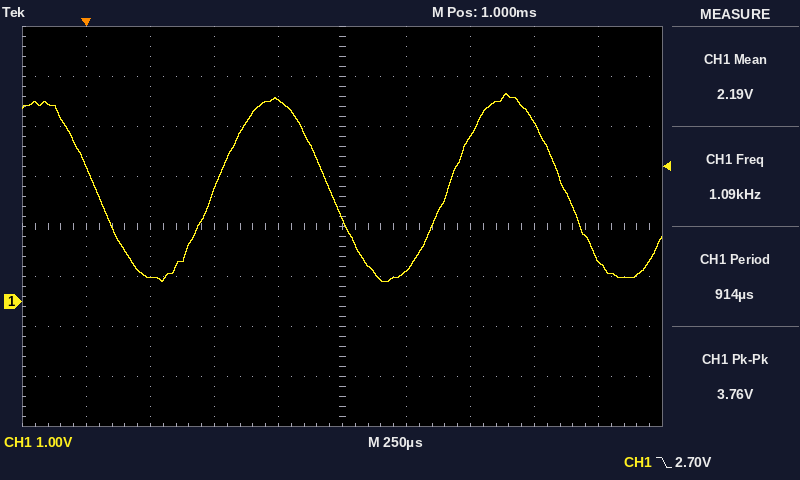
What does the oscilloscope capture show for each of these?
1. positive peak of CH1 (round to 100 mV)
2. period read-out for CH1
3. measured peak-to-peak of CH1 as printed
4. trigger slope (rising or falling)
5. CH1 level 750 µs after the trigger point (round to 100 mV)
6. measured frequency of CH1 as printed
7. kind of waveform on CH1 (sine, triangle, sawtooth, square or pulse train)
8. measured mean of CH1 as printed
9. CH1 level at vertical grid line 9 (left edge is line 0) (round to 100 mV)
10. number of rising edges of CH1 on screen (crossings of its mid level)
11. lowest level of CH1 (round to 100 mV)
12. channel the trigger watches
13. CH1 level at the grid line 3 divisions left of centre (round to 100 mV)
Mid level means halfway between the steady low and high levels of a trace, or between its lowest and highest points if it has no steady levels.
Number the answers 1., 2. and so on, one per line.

1. 4.2 V
2. 914 µs
3. 3.76 V
4. falling
5. 4.0 V
6. 1.09 kHz
7. sine
8. 2.19 V
9. 800 mV
10. 2
11. 400 mV
12. CH1
13. 500 mV
